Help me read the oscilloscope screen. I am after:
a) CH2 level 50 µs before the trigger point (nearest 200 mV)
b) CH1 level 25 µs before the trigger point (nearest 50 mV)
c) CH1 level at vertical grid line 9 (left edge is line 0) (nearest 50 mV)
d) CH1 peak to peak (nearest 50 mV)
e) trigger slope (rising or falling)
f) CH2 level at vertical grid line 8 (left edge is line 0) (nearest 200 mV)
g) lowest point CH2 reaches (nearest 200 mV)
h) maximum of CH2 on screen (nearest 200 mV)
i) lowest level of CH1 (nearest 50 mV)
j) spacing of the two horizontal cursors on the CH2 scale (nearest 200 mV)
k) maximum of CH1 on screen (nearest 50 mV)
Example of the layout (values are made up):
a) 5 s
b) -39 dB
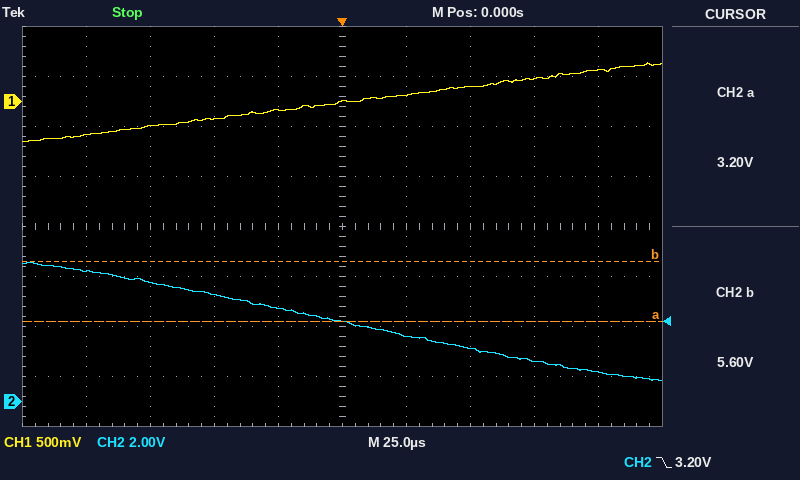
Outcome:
a) 4.2 V
b) -100 mV
c) 300 mV
d) 800 mV
e) falling
f) 1.6 V
g) 800 mV
h) 5.6 V
i) -400 mV
j) 2.4 V
k) 400 mV
